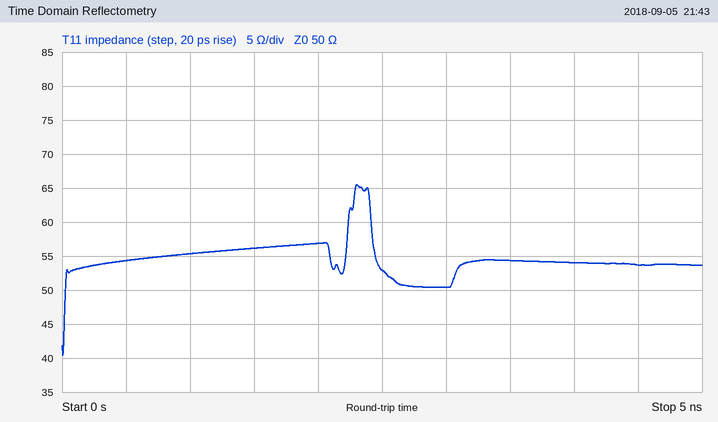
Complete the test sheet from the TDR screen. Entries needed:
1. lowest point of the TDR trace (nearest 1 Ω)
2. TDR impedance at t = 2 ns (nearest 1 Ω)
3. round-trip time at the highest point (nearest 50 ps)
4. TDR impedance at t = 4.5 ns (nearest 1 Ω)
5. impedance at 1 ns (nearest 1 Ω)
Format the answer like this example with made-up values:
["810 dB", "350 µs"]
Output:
["40 Ω", "57 Ω", "2.30 ns", "54 Ω", "55 Ω"]
